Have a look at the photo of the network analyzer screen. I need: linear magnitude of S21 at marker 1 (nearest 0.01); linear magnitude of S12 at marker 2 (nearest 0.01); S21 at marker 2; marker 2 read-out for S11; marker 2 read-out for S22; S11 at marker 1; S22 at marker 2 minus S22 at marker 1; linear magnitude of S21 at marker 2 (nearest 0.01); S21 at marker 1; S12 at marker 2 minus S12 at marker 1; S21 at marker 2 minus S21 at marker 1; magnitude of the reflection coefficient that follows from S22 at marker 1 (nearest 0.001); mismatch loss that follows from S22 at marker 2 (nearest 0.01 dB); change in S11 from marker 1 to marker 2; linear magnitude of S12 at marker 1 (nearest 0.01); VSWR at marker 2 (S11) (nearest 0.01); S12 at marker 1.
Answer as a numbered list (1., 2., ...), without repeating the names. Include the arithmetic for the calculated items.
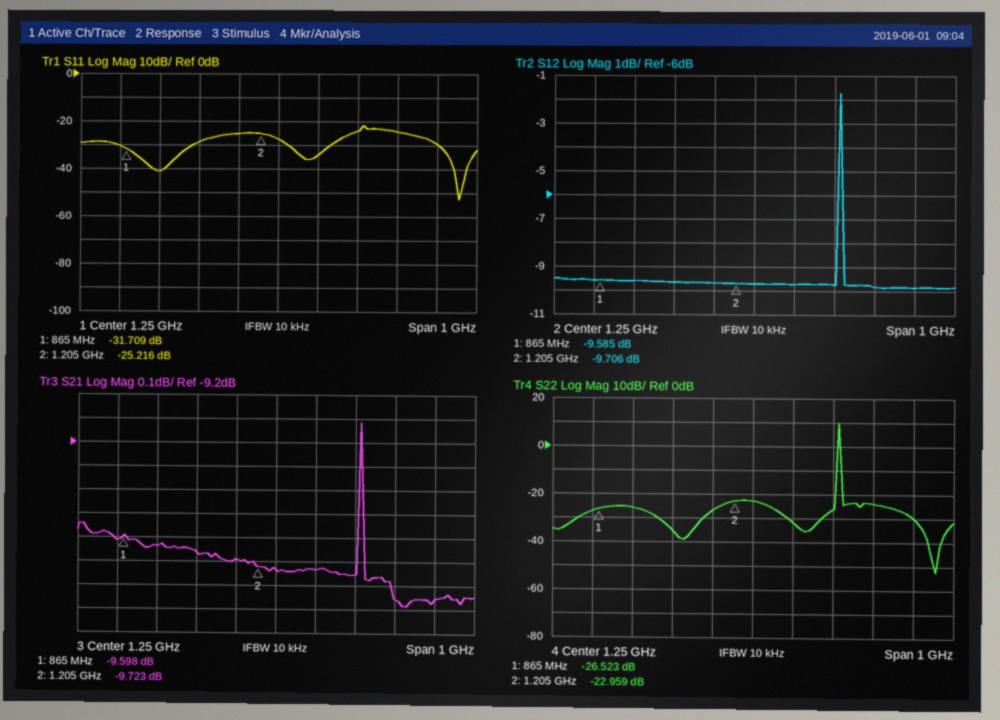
1. 10^(-9.598/20) ≈ 0.33
2. 10^(-9.706/20) ≈ 0.33
3. -9.723 dB
4. -25.216 dB
5. -22.959 dB
6. -31.709 dB
7. -22.959 − (-26.523) = 3.564 dB
8. 10^(-9.723/20) ≈ 0.33
9. -9.598 dB
10. -9.706 − (-9.585) = -0.121 dB
11. -9.723 − (-9.598) = -0.125 dB
12. 10^(-26.523/20) ≈ 0.047
13. −10 log10(1 − 10^(-22.959/10)) ≈ 0.02 dB
14. -25.216 − (-31.709) = 6.493 dB
15. 10^(-9.585/20) ≈ 0.33
16. (1 + 0.0549)/(1 − 0.0549) ≈ 1.12
17. -9.585 dB
